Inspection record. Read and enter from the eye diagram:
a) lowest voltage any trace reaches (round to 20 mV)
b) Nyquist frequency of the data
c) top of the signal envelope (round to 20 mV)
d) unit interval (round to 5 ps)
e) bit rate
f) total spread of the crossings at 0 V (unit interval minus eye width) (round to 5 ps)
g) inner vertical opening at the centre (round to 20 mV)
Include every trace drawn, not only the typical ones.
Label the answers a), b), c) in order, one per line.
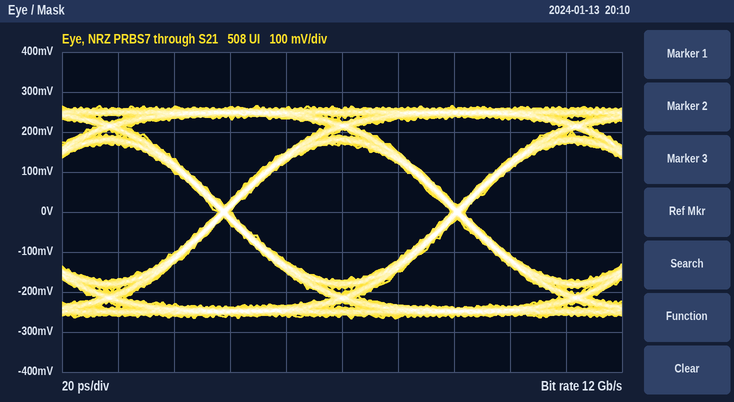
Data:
a) -260 mV
b) 6 GHz
c) 260 mV
d) 85 ps
e) 12 Gb/s
f) 5 ps
g) 340 mV
